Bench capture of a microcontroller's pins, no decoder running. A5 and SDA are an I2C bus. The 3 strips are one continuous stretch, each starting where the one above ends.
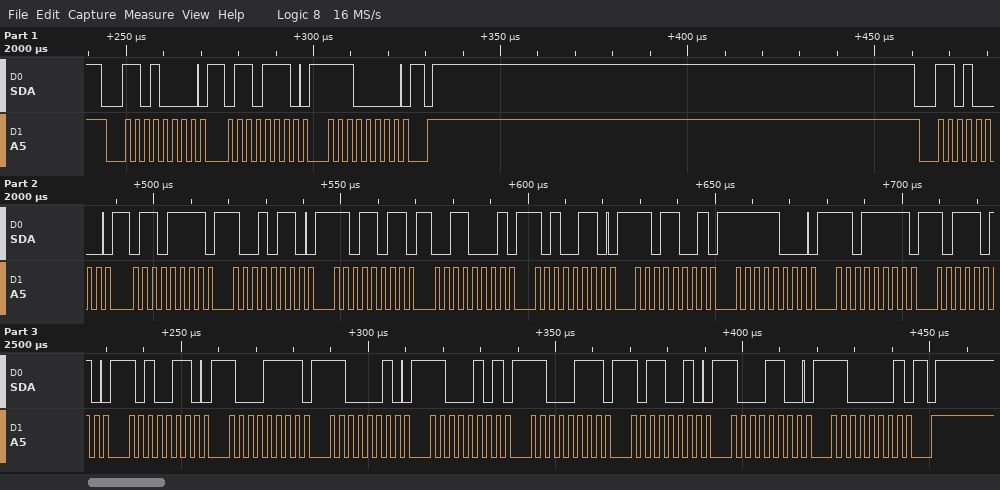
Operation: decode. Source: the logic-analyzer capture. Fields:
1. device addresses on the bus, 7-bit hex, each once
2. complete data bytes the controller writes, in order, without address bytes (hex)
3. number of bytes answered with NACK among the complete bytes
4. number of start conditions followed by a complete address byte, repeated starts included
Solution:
0x68
6E E0 6F 96 DB 31 A6 D9 F8 DF BA A6 8F C2 C5 C7 B2 8C C1
0
2
